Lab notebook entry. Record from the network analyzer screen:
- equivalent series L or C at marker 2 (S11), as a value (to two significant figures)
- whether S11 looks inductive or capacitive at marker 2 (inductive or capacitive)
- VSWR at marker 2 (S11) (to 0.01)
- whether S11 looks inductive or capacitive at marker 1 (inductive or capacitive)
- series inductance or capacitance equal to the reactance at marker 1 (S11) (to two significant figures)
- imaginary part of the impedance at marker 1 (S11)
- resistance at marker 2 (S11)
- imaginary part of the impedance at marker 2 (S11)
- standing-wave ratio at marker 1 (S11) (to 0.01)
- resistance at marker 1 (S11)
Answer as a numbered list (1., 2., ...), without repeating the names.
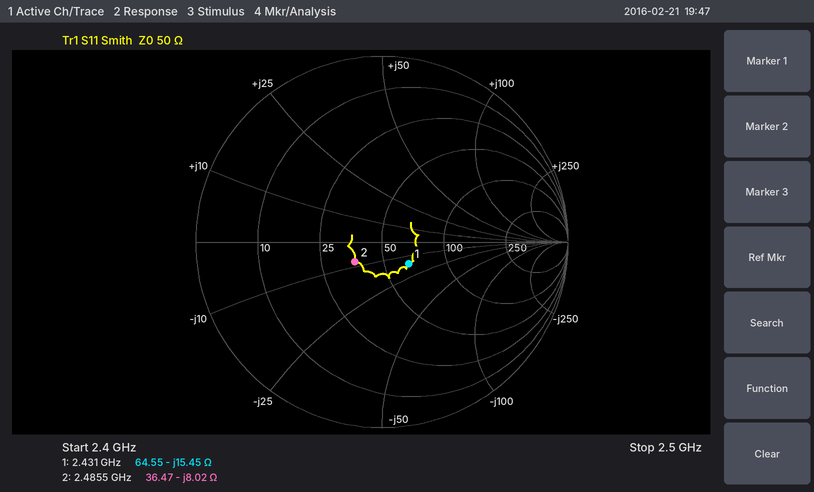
1. 8.0 pF
2. capacitive
3. 1.44
4. capacitive
5. 4.2 pF
6. -15.45 Ω
7. 36.47 Ω
8. -8.02 Ω
9. 1.45
10. 64.55 Ω
